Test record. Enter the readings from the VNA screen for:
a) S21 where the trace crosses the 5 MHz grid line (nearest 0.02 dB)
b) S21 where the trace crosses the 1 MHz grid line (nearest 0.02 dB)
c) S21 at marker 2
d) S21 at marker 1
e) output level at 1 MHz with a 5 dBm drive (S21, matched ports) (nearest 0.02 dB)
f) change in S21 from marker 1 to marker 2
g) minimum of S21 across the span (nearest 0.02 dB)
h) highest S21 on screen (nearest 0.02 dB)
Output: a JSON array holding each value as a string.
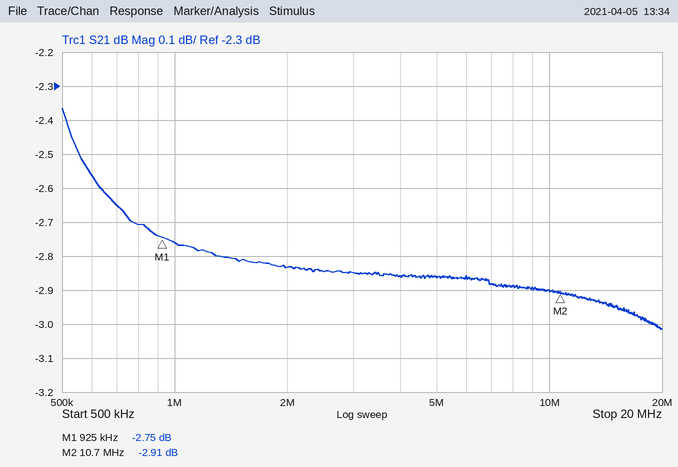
["-2.86 dB", "-2.76 dB", "-2.91 dB", "-2.75 dB", "2.24 dBm", "-0.16 dB", "-3.02 dB", "-2.36 dB"]
